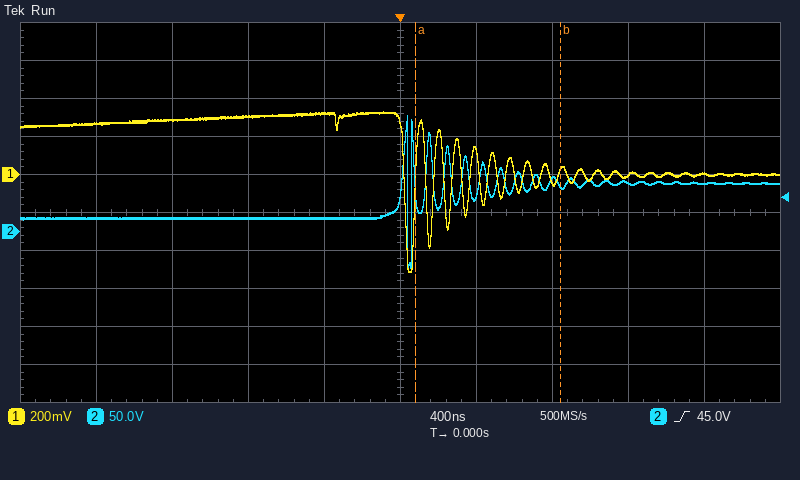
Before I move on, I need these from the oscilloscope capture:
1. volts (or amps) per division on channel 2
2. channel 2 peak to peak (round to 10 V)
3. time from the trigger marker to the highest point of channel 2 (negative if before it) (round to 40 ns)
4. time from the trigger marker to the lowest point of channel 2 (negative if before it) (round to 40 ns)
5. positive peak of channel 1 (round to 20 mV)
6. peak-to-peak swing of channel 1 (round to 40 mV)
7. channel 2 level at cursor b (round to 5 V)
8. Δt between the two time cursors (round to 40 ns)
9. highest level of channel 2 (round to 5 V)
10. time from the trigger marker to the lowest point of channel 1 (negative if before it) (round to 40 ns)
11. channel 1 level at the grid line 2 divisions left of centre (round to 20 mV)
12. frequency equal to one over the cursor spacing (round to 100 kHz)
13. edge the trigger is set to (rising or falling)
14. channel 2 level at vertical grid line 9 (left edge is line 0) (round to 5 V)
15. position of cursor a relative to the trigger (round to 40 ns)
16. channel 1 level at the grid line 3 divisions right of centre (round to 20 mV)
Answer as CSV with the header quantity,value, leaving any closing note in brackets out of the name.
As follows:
quantity,value
volts (or amps) per division on channel 2,50 V
channel 2 peak to peak,200 V
time from the trigger marker to the highest point of channel 2 (negative if before it),+40 ns
time from the trigger marker to the lowest point of channel 2 (negative if before it),+40 ns
positive peak of channel 1,340 mV
peak-to-peak swing of channel 1,840 mV
channel 2 level at cursor b,60 V
Δt between the two time cursors,760 ns
highest level of channel 2,155 V
time from the trigger marker to the lowest point of channel 1 (negative if before it),+40 ns
channel 1 level at the grid line 2 divisions left of centre,300 mV
frequency equal to one over the cursor spacing,1.3 MHz
edge the trigger is set to,rising
channel 2 level at vertical grid line 9 (left edge is line 0),65 V
position of cursor a relative to the trigger,+80 ns
channel 1 level at the grid line 3 divisions right of centre,0 mV
